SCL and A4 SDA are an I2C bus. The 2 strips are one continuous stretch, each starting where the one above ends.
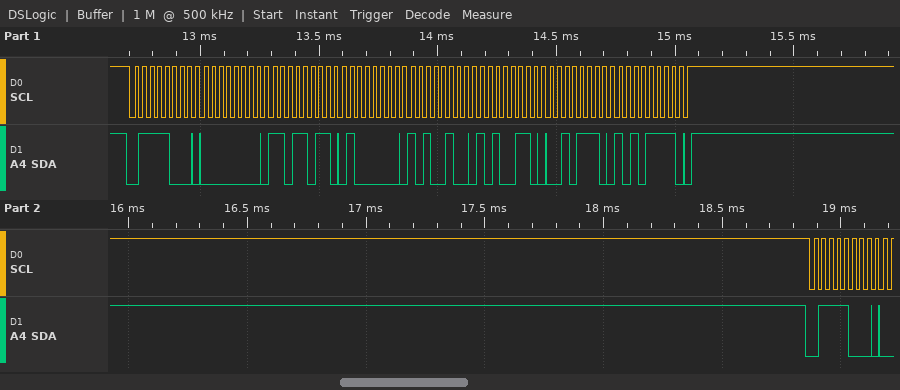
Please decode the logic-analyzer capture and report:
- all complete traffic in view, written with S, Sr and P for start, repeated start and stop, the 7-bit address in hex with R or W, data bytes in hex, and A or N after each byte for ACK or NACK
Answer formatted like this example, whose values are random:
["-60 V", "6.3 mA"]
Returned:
["S 3CW A 00 A DB A 40 A A4 A A6 A 2E A AF A P S 3CW A"]
